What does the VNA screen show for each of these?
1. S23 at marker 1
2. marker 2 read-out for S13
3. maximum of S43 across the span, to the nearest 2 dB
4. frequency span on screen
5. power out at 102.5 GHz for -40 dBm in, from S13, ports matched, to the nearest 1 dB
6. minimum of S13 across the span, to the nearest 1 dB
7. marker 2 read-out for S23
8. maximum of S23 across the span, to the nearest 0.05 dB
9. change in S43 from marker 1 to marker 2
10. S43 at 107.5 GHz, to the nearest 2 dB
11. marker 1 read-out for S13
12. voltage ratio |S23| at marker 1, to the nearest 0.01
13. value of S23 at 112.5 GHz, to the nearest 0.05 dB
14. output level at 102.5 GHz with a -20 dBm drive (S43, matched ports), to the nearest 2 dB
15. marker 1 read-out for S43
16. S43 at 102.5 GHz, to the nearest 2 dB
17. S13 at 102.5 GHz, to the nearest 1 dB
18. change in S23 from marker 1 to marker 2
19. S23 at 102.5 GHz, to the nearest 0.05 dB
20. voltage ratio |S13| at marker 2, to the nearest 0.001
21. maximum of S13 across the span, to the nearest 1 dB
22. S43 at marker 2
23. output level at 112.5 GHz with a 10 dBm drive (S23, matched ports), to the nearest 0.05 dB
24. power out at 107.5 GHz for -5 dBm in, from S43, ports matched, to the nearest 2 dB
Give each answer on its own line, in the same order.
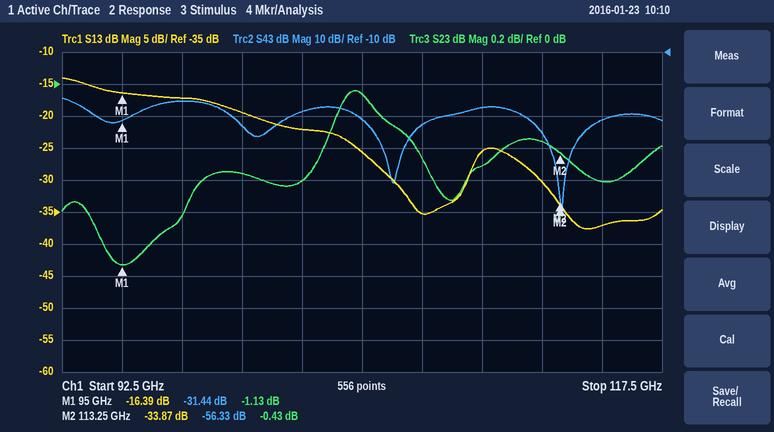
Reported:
-1.13 dB
-33.87 dB
-24 dB
25 GHz
-62 dBm
-38 dB
-0.43 dB
-0.05 dB
-24.89 dB
-32 dB
-16.39 dB
0.88
-0.35 dB
-48 dBm
-31.44 dB
-28 dB
-22 dB
0.70 dB
-0.60 dB
0.020
-14 dB
-56.33 dB
9.65 dBm
-38 dBm
